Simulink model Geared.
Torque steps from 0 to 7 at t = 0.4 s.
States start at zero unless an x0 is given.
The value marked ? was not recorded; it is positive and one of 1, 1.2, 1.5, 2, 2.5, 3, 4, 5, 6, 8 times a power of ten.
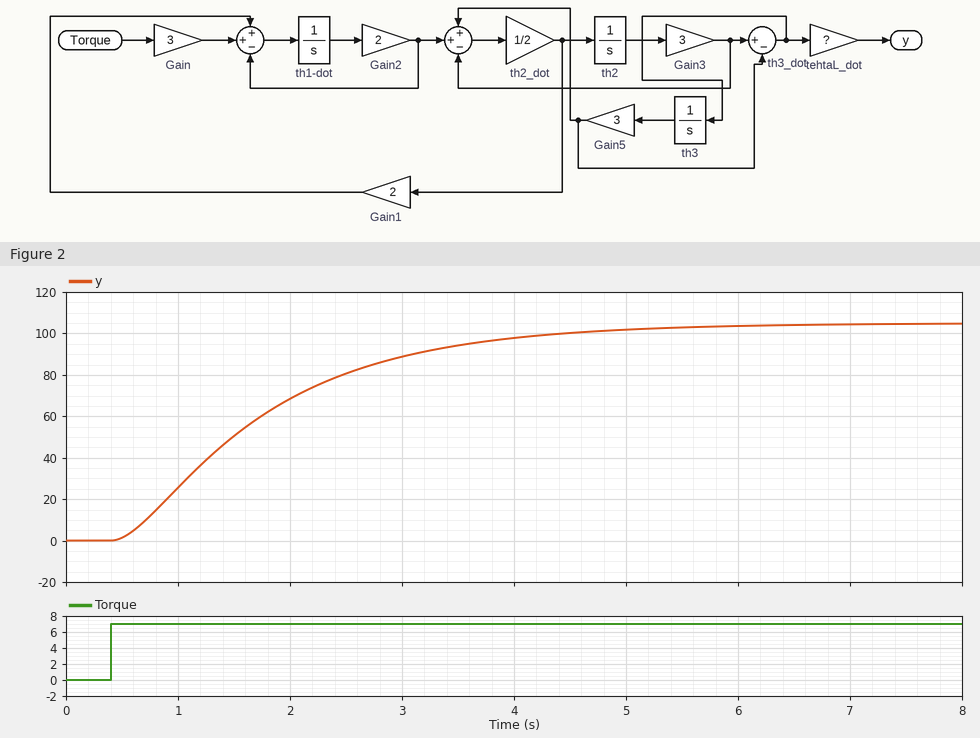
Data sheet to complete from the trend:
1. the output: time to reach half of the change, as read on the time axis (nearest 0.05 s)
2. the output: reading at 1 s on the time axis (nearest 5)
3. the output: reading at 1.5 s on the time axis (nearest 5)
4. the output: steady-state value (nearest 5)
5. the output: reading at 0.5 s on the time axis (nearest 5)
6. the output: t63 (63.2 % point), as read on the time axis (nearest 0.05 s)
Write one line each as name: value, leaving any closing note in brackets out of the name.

the output: time to reach half of the change, as read on the time axis: 1.55 s
the output: reading at 1 s on the time axis: 25
the output: reading at 1.5 s on the time axis: 50
the output: steady-state value: 105
the output: reading at 0.5 s on the time axis: 0
the output: t63 (63.2 % point), as read on the time axis: 1.95 s
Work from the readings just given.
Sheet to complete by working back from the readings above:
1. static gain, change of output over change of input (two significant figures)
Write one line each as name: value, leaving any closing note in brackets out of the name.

static gain, change of output over change of input: 15
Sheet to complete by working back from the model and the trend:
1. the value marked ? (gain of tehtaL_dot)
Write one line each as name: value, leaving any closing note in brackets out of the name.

the value marked ?: 5
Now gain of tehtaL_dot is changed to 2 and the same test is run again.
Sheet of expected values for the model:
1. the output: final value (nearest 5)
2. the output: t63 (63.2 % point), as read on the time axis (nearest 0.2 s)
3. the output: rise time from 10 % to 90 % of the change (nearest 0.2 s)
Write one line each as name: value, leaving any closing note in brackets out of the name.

the output: final value: 40
the output: t63 (63.2 % point), as read on the time axis: 2.0 s
the output: rise time from 10 % to 90 % of the change: 2.8 s
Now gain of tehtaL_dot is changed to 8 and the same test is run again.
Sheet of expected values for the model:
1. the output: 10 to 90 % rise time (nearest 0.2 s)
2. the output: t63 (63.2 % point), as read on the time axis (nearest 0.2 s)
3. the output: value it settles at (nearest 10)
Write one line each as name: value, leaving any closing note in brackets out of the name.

the output: 10 to 90 % rise time: 2.8 s
the output: t63 (63.2 % point), as read on the time axis: 2.0 s
the output: value it settles at: 170
